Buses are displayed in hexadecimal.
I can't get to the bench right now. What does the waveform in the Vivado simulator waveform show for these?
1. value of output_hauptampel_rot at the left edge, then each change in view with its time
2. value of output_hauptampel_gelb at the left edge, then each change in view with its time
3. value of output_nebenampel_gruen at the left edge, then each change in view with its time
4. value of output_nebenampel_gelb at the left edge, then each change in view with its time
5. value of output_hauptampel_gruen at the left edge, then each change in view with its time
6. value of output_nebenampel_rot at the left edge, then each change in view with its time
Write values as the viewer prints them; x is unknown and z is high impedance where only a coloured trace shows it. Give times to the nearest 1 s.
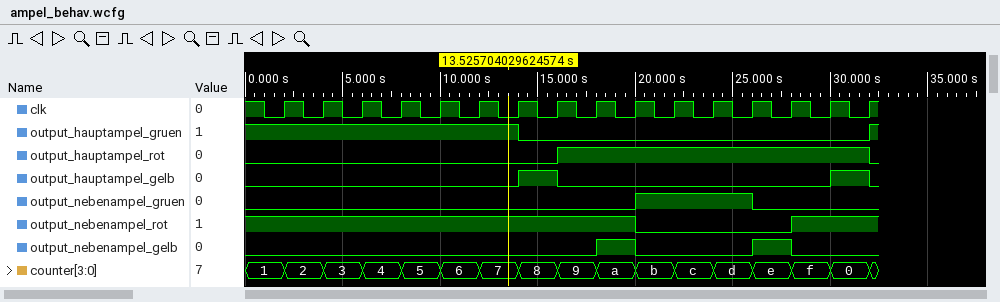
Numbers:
0, 1 at 16 s, 0 at 32 s
0, 1 at 14 s, 0 at 16 s, 1 at 30 s, 0 at 32 s
0, 1 at 20 s, 0 at 26 s
0, 1 at 18 s, 0 at 20 s, 1 at 26 s, 0 at 28 s
1, 0 at 14 s, 1 at 32 s
1, 0 at 20 s, 1 at 28 s
